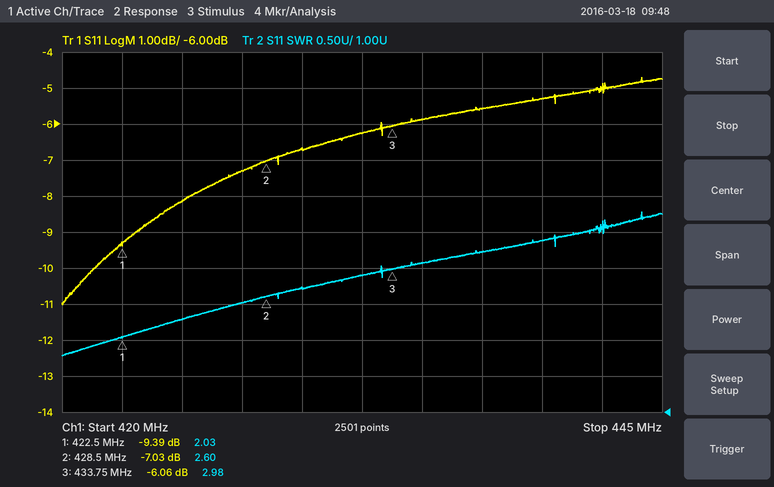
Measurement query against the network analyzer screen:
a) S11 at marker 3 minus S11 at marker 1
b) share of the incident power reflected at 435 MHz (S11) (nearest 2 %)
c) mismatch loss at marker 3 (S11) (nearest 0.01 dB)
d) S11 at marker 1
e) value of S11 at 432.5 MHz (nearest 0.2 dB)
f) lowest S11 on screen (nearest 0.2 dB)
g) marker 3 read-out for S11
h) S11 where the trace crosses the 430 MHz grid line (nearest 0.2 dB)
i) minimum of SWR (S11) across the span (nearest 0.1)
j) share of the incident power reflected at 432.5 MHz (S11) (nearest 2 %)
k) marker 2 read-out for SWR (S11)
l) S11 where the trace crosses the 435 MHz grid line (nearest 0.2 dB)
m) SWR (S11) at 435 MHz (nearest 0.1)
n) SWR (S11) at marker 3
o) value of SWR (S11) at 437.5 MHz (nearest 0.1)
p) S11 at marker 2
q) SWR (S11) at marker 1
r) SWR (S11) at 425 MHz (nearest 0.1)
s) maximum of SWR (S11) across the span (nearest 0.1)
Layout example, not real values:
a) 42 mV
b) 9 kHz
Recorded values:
a) 3.33 dB
b) 26 %
c) 1.24 dB
d) -9.39 dB
e) -6.2 dB
f) -11.0 dB
g) -6.06 dB
h) -6.6 dB
i) 1.8
j) 24 %
k) 2.60
l) -5.8 dB
m) 3.1
n) 2.98
o) 3.2
p) -7.03 dB
q) 2.03
r) 2.3
s) 3.8
